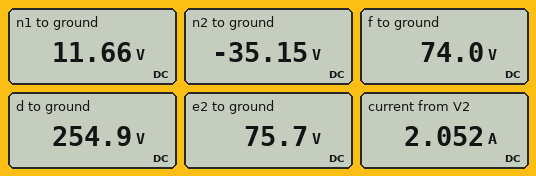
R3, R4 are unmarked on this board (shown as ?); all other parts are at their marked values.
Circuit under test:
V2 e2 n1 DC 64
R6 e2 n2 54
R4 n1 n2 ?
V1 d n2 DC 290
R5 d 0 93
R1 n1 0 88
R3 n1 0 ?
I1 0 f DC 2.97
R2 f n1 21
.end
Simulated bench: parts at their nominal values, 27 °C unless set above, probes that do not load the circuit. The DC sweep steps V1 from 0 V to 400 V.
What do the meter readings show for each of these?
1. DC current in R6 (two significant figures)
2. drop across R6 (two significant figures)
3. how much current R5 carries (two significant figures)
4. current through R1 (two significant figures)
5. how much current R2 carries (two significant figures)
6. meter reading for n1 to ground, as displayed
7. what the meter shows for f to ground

2.1 A
110 V
2.7 A
130 mA
3.0 A
11.66 V
74.0 V
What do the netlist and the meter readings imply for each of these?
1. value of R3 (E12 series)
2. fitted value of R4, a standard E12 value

120 Ω
68 Ω
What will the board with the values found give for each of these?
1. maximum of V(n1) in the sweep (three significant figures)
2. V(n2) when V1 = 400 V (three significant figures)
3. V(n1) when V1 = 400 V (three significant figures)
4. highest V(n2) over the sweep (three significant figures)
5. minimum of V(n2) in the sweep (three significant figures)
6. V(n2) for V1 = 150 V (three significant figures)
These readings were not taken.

96.3 V
-86.3 V
-20.5 V
99.7 V
-86.3 V
30.0 V
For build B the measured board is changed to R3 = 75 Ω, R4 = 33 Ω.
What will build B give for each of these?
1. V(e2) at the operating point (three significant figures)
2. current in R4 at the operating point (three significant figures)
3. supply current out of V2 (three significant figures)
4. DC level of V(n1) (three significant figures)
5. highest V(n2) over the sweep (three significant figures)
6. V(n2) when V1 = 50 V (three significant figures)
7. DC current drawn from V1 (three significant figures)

70.0 V
1.02 A
1.81 A
5.99 V
87.3 V
67.5 V
2.82 A
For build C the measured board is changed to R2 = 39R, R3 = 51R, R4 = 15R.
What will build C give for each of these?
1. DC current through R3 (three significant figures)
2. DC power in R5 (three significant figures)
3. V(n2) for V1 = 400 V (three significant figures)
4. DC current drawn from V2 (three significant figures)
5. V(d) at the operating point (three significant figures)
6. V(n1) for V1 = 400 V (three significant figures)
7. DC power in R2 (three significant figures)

33.1 mA
792 W
-54.0 V
1.56 A
271 V
-24.2 V
344 W
